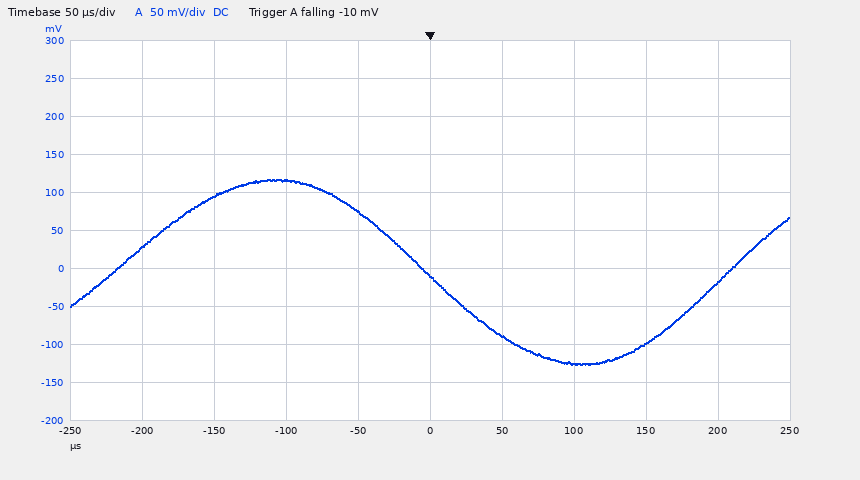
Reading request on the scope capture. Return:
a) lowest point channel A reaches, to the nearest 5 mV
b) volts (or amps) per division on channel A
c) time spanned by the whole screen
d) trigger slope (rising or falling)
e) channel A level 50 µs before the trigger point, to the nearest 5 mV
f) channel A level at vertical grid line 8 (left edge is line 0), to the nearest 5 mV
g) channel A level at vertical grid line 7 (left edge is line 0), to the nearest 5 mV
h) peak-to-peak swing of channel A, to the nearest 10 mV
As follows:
-125 mV
50 mV
500 µs
falling
75 mV
-100 mV
-125 mV
240 mV
